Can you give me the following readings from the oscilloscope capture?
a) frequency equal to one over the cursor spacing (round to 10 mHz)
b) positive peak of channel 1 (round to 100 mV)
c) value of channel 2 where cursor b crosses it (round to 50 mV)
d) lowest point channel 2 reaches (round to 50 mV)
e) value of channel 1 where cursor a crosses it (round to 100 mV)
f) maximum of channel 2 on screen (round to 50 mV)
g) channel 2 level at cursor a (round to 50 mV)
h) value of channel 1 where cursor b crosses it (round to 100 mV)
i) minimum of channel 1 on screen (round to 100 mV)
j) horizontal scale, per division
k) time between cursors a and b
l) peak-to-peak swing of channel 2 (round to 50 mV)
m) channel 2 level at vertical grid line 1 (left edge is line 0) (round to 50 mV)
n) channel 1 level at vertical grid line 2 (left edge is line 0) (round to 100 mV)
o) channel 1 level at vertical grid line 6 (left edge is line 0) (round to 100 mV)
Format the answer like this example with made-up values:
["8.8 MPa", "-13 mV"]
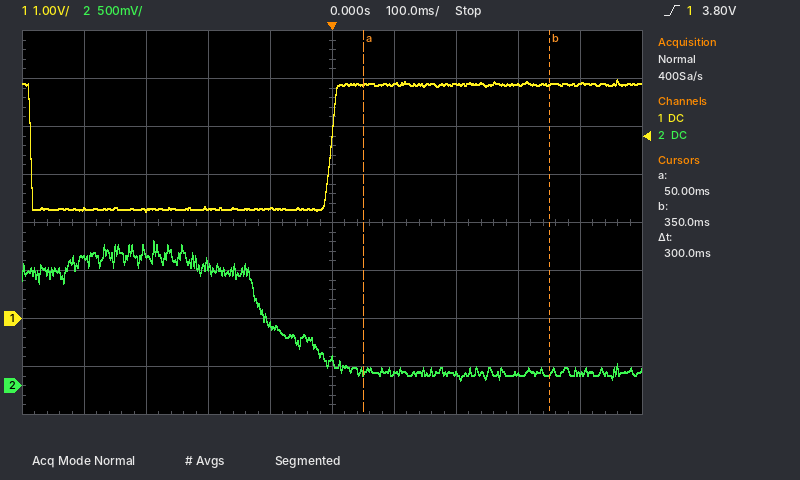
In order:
["3.33 Hz", "5.0 V", "150 mV", "50 mV", "4.9 V", "1.50 V", "150 mV", "4.9 V", "2.2 V", "100 ms", "300 ms", "1.45 V", "1.35 V", "2.3 V", "4.9 V"]
